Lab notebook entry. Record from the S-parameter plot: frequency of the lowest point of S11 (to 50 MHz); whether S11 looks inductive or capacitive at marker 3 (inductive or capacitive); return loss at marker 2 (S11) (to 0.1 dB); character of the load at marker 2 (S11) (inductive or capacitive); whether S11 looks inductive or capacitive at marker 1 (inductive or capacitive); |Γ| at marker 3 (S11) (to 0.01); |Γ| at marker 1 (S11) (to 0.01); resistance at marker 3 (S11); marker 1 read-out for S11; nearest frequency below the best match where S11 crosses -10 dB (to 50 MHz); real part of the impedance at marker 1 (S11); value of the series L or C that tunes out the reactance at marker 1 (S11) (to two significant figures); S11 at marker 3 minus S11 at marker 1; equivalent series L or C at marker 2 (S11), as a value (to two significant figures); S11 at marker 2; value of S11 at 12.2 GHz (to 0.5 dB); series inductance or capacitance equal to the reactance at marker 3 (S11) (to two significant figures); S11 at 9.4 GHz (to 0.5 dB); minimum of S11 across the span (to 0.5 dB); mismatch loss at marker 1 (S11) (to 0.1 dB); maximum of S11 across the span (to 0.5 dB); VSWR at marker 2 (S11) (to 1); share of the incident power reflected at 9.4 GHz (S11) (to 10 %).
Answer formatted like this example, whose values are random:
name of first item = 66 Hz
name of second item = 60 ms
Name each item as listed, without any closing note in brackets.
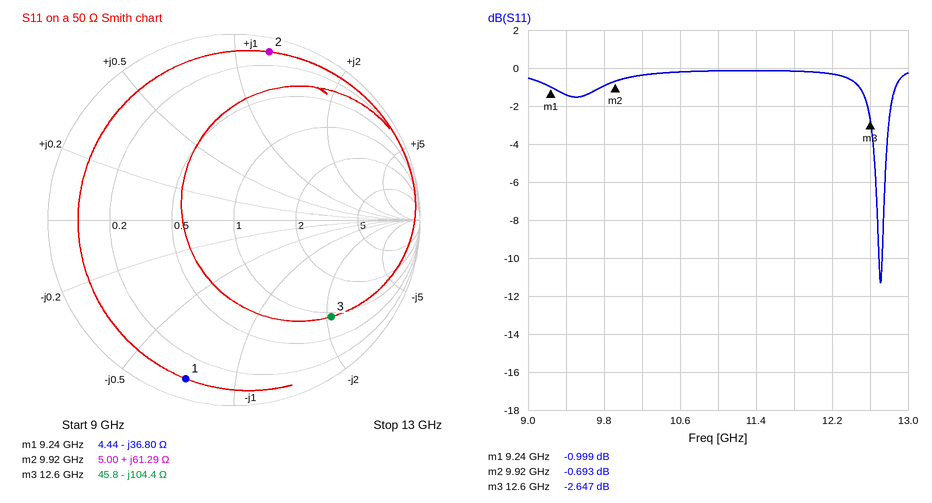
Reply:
frequency of the lowest point of S11 = 12.70 GHz
whether S11 looks inductive or capacitive at marker 3 = capacitive
return loss at marker 2 (S11) = 0.7 dB
character of the load at marker 2 (S11) = inductive
whether S11 looks inductive or capacitive at marker 1 = capacitive
|Γ| at marker 3 (S11) = 0.74
|Γ| at marker 1 (S11) = 0.89
resistance at marker 3 = 45.8 Ω
marker 1 read-out for S11 = -0.999 dB
nearest frequency below the best match where S11 crosses -10 dB = 12.70 GHz
real part of the impedance at marker 1 = 4.44 Ω
value of the series L or C that tunes out the reactance at marker 1 (S11) = 630 pH
S11 at marker 3 minus S11 at marker 1 = -1.648 dB
equivalent series L or C at marker 2 (S11), as a value = 980 pH
S11 at marker 2 = -0.693 dB
value of S11 at 12.2 GHz = -0.5 dB
series inductance or capacitance equal to the reactance at marker 3 (S11) = 120 fF
S11 at 9.4 GHz = -1.5 dB
minimum of S11 across the span = -11.5 dB
mismatch loss at marker 1 (S11) = 6.9 dB
maximum of S11 across the span = 0.0 dB
VSWR at marker 2 (S11) = 25
share of the incident power reflected at 9.4 GHz (S11) = 70 %
